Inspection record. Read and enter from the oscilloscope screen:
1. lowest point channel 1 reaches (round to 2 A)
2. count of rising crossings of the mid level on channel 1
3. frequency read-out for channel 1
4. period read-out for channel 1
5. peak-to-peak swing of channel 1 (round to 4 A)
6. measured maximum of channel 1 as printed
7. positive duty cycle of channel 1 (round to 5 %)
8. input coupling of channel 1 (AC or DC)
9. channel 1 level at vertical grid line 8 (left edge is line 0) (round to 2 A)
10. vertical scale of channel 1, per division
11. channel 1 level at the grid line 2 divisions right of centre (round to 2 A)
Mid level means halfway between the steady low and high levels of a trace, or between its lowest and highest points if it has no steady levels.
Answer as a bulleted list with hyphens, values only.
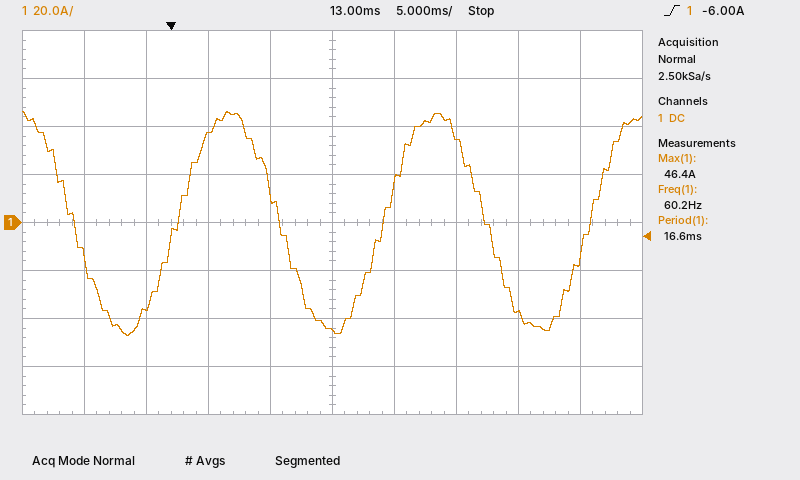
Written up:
- -48 A
- 3
- 60.2 Hz
- 16.6 ms
- 92 A
- 46.4 A
- 50 %
- DC
- -38 A
- 20 A
- 36 A
